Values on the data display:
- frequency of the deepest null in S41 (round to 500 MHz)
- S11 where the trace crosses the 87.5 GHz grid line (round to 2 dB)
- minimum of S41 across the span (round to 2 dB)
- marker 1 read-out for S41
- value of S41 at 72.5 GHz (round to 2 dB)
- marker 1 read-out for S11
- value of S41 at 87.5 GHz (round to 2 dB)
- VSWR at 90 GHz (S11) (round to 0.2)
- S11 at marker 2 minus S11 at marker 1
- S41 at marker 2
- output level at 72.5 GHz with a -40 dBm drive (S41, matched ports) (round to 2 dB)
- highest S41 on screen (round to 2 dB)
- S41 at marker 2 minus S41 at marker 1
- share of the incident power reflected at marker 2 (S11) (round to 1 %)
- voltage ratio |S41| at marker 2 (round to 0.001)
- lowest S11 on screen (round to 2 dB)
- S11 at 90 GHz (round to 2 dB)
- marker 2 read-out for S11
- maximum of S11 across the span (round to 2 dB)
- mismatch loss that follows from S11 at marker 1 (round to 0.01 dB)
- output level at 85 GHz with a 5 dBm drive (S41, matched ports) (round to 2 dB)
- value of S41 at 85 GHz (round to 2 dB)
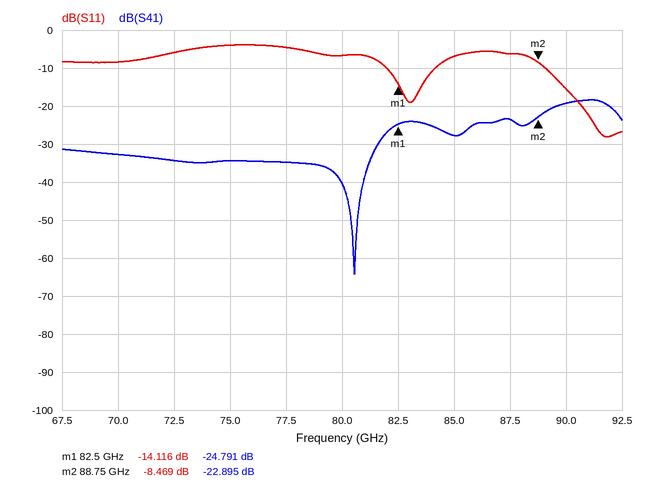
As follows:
80.5 GHz
-6 dB
-64 dB
-24.791 dB
-34 dB
-14.116 dB
-24 dB
1.4
5.647 dB
-22.895 dB
-74 dBm
-18 dB
1.896 dB
14 %
0.072
-28 dB
-16 dB
-8.469 dB
-4 dB
0.17 dB
-22 dBm
-28 dB
